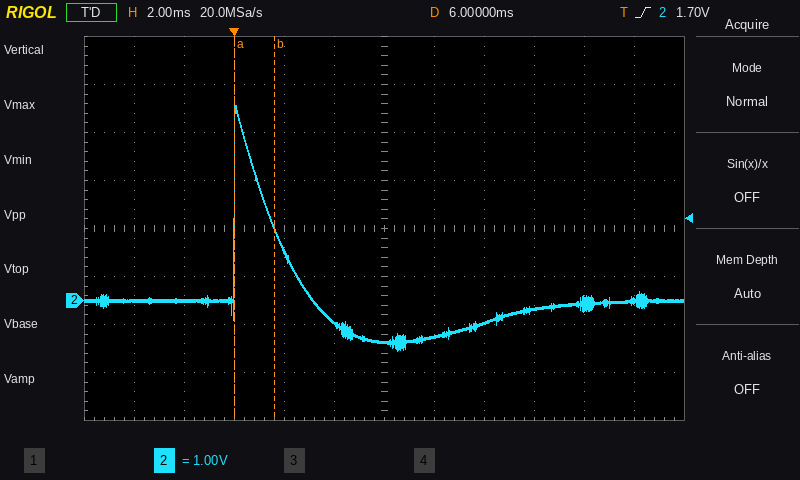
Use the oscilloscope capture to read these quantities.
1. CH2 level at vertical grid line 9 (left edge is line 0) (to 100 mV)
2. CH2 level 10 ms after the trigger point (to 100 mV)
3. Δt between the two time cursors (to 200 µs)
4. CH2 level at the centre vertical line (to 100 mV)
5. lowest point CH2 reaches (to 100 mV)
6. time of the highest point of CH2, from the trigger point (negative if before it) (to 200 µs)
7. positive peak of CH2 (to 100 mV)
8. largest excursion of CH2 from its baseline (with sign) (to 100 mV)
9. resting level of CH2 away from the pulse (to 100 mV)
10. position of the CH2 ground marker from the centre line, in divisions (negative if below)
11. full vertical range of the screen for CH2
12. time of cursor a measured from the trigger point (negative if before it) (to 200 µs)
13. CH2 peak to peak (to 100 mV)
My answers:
-200 mV
-500 mV
1.6 ms
-900 mV
-1.0 V
0.0 ms
4.1 V
+4.1 V
0.0 V
-1.5 div
8 V
0.0 ms
5.1 V
